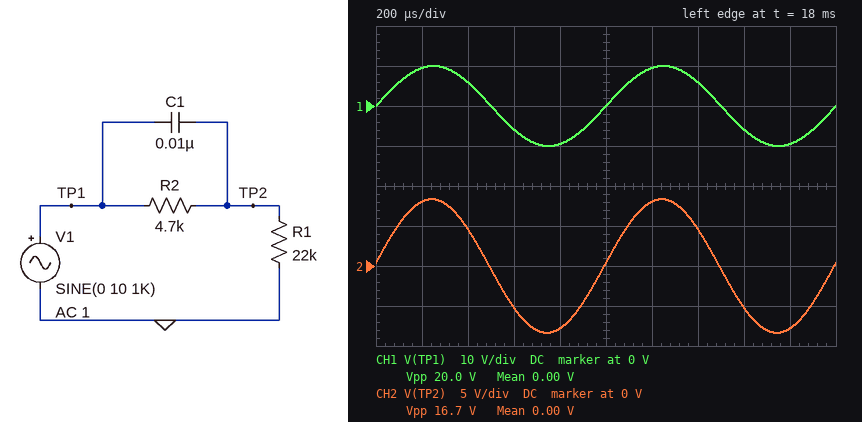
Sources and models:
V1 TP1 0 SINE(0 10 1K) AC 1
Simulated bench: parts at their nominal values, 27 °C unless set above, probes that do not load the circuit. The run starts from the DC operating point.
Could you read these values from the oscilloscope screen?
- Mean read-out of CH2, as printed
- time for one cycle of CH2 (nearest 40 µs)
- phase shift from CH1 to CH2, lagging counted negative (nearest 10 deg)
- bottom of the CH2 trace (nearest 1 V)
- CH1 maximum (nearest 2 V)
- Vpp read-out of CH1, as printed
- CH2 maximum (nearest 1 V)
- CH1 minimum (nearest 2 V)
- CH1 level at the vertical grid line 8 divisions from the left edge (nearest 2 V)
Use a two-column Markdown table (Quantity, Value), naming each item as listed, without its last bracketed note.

| Quantity | Value |
|---|---|
| Mean read-out of CH2, as printed | 0.00 V |
| time for one cycle of CH2 | 1.00 ms |
| phase shift from CH1 to CH2, lagging counted negative | 0 deg |
| bottom of the CH2 trace | -8 V |
| CH1 maximum | 10 V |
| Vpp read-out of CH1, as printed | 20.0 V |
| CH2 maximum | 8 V |
| CH1 minimum | -10 V |
| CH1 level at the vertical grid line 8 divisions from the left edge | -6 V |
